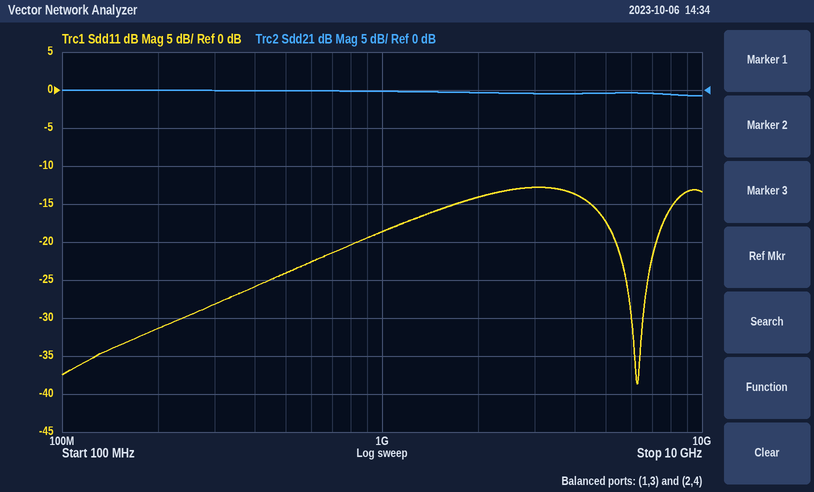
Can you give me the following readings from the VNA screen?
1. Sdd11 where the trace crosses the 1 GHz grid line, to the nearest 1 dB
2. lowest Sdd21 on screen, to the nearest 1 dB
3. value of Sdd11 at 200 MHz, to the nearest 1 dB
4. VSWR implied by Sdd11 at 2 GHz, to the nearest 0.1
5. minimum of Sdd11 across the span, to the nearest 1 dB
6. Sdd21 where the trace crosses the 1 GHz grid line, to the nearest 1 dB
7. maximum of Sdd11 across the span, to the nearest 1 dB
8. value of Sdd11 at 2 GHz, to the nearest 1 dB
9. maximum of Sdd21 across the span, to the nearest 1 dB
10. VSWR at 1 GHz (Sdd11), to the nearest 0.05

-19 dB
-1 dB
-31 dB
1.5
-39 dB
0 dB
-13 dB
-14 dB
0 dB
1.25
